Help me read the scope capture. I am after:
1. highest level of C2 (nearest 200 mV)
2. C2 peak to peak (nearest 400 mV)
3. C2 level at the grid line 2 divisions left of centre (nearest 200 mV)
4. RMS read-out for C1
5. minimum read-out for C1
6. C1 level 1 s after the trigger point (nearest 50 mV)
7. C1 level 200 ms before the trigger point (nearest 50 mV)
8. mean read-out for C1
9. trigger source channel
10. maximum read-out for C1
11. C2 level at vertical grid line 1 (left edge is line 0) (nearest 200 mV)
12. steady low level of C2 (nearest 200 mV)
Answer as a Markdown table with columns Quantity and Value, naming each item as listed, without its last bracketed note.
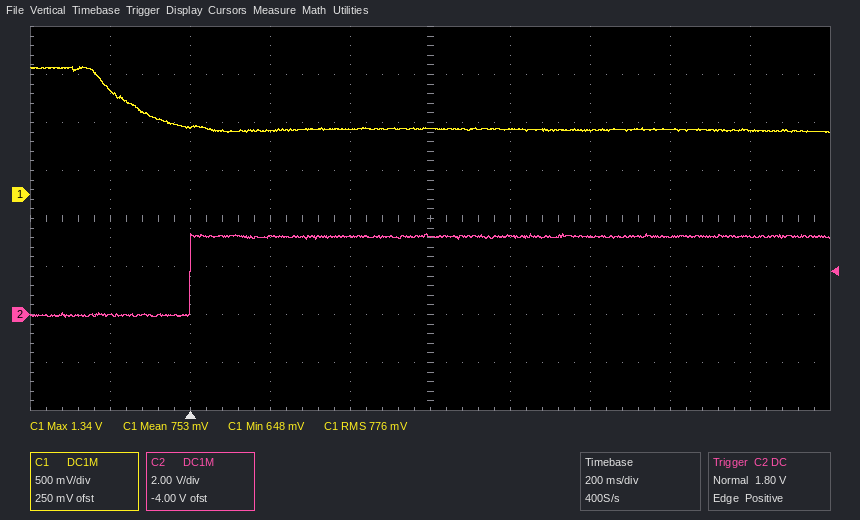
| Quantity | Value |
|---|---|
| highest level of C2 | 3.4 V |
| C2 peak to peak | 3.6 V |
| C2 level at the grid line 2 divisions left of centre | 3.2 V |
| RMS read-out for C1 | 776 mV |
| minimum read-out for C1 | 648 mV |
| C1 level 1 s after the trigger point | 650 mV |
| C1 level 200 ms before the trigger point | 1.10 V |
| mean read-out for C1 | 753 mV |
| trigger source channel | C2 |
| maximum read-out for C1 | 1.34 V |
| C2 level at vertical grid line 1 (left edge is line 0) | 0.0 V |
| steady low level of C2 | 0.0 V |
